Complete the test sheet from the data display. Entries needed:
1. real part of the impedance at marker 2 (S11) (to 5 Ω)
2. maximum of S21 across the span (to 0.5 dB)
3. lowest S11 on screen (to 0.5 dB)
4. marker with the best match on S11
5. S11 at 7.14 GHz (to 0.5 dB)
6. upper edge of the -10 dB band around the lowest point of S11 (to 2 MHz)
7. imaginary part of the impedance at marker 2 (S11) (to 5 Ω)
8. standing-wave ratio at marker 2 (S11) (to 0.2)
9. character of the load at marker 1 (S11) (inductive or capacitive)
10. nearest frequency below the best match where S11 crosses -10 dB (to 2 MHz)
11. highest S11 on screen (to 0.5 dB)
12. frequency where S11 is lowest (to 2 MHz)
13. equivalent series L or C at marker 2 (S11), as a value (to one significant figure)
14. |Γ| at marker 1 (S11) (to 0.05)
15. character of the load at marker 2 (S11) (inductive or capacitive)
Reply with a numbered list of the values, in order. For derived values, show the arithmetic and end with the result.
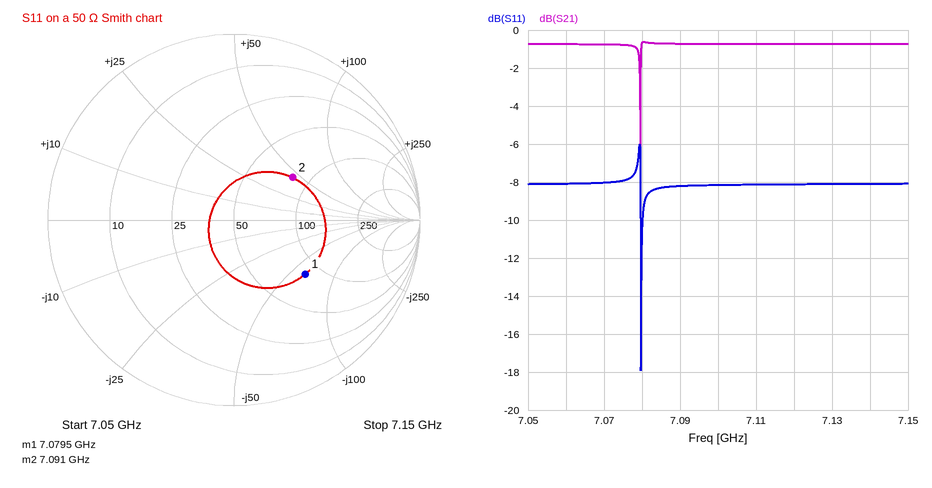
1. 80 Ω
2. -0.5 dB
3. -18.0 dB
4. marker 2
5. -8.0 dB
6. 7.080 GHz
7. +45 Ω
8. 2.2
9. capacitive
10. 7.080 GHz
11. -6.0 dB
12. 7.080 GHz
13. L = 45 Ω/(2π × 7.091 GHz) ≈ 1.0 nH
14. 0.50
15. inductive
